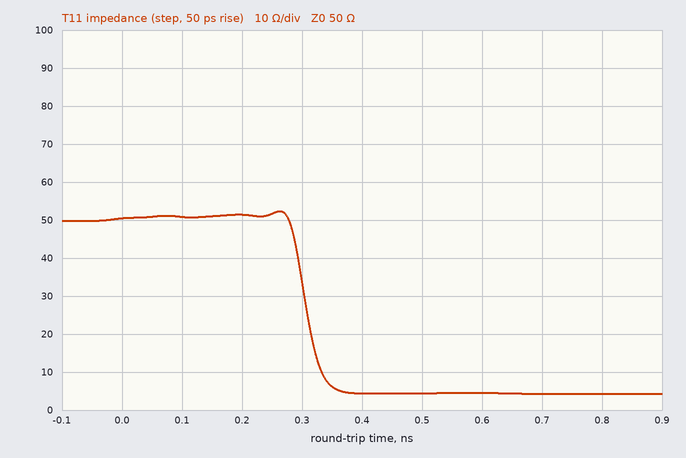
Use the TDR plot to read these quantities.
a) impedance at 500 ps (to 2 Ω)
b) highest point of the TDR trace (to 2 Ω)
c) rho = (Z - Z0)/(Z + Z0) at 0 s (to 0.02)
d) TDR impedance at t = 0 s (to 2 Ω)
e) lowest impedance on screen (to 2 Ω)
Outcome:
4 Ω
52 Ω
0.00
50 Ω
4 Ω
